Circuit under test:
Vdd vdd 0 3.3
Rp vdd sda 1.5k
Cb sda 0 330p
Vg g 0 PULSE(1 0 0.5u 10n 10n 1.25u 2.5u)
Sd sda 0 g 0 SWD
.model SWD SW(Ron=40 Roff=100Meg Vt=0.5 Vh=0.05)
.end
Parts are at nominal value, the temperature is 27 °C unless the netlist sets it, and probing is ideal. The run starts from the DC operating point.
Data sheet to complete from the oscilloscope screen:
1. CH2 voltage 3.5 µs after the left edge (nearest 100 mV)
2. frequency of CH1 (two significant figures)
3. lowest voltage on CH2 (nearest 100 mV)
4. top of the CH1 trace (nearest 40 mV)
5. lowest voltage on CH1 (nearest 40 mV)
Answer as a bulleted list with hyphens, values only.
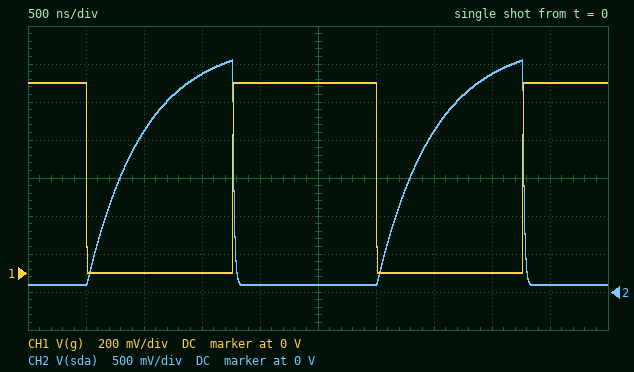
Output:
- 2.1 V
- 400 kHz
- 100 mV
- 1.00 V
- 0 V
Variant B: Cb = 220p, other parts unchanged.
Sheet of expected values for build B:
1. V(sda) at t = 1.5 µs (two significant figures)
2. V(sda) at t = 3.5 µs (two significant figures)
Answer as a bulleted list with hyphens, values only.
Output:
- 3.1 V
- 2.6 V
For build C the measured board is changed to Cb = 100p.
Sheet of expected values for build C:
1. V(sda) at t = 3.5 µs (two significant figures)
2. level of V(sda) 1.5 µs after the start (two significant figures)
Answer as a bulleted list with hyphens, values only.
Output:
- 3.2 V
- 3.3 V
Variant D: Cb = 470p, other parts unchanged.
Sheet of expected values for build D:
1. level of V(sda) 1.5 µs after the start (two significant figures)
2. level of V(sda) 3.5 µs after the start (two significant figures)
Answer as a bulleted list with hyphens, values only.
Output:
- 2.5 V
- 1.7 V
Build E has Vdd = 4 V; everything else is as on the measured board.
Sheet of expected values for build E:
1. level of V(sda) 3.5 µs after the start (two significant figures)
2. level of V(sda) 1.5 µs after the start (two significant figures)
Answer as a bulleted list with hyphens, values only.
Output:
- 2.6 V
- 3.5 V
